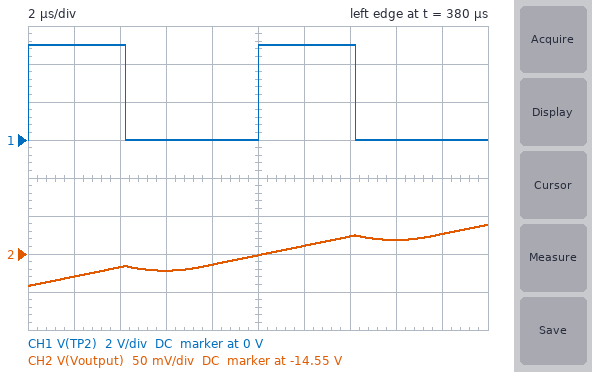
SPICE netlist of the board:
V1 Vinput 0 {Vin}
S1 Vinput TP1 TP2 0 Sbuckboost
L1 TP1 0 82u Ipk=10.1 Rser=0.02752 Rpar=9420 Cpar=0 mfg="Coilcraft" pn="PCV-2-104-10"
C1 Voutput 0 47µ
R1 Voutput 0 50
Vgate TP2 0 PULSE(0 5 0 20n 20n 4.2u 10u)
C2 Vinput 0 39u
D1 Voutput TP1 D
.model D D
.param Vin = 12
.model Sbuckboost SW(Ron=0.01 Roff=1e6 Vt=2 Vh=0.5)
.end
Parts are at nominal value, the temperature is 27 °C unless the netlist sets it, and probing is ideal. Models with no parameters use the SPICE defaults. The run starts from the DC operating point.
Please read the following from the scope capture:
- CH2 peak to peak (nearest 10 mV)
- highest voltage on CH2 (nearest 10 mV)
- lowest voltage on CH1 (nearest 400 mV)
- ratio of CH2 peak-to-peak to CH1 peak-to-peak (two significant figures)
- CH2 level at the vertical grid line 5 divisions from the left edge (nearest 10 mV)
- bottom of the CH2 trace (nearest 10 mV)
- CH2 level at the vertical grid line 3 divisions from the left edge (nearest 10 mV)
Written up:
80 mV
-14.51 V
0 V
0.016
-14.55 V
-14.59 V
-14.57 V
